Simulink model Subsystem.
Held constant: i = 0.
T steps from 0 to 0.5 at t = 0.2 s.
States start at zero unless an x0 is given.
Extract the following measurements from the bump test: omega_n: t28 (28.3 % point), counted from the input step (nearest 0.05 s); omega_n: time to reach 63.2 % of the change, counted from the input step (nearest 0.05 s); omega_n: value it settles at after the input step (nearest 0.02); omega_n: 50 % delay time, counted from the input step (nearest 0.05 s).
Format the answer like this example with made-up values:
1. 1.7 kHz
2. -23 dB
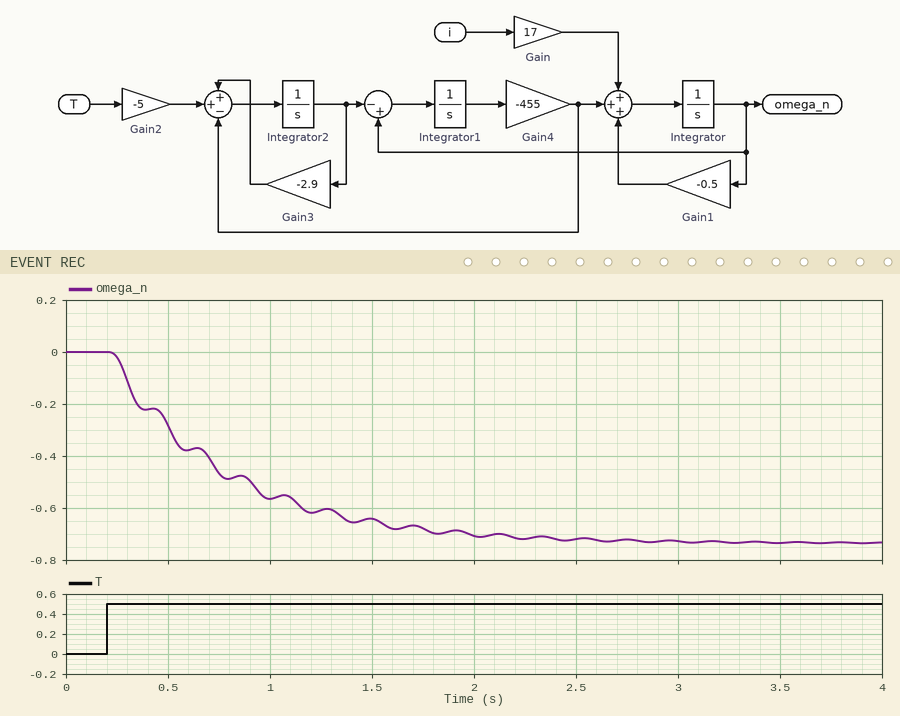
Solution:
1. 0.15 s
2. 0.55 s
3. -0.74
4. 0.35 s
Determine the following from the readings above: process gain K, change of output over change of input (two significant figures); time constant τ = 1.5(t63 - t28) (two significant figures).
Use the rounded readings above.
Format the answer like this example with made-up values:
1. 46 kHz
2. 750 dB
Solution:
1. -1.5
2. 0.60 s
